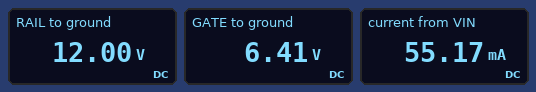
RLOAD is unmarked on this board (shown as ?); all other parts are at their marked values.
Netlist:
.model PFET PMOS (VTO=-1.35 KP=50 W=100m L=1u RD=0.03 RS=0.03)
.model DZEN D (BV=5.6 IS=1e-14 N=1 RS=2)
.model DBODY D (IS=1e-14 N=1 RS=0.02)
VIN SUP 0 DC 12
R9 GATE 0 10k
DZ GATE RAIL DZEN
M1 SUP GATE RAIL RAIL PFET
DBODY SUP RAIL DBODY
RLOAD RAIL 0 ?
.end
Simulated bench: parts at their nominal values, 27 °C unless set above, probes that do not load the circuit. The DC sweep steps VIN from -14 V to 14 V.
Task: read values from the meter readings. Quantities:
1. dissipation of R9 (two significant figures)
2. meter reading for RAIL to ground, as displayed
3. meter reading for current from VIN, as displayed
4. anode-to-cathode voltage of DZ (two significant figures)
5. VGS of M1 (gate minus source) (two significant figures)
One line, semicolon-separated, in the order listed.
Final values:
4.1 mW; 12.00 V; 55.17 mA; -5.6 V; -5.6 V
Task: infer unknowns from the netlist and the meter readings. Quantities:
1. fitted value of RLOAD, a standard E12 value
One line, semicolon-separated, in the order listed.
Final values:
220 Ω
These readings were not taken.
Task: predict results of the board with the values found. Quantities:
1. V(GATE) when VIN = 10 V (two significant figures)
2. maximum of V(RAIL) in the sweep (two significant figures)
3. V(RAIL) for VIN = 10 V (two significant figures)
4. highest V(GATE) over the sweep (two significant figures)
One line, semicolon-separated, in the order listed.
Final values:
4.4 V; 14 V; 10 V; 8.4 V
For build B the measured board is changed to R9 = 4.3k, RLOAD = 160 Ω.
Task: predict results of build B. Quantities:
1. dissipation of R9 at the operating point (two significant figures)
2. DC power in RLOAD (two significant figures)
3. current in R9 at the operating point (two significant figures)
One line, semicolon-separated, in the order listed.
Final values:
9.5 mW; 900 mW; 1.5 mA
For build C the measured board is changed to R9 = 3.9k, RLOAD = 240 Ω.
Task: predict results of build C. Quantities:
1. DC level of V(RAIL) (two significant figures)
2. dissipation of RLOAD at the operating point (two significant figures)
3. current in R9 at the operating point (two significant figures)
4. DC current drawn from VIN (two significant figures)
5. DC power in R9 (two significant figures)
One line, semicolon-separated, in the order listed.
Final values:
12 V; 600 mW; 1.6 mA; 52 mA; 10 mW
